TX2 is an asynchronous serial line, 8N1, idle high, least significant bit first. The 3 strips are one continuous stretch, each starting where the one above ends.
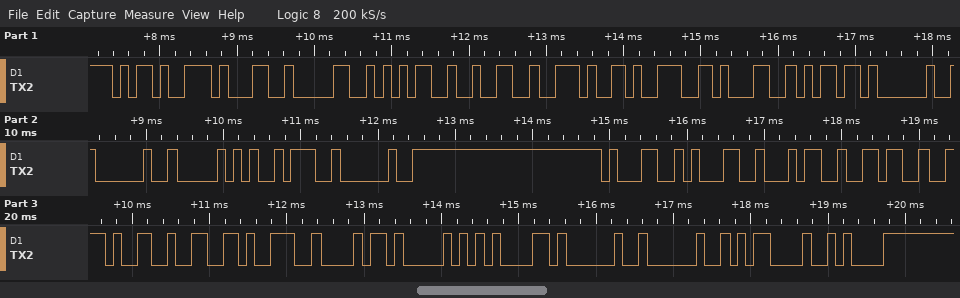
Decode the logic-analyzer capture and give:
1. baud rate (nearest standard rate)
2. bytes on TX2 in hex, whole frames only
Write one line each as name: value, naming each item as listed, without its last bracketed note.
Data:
baud rate: 9600 baud
bytes on TX2 in hex, whole frames only: 2D 31 30 35 32 2E 39 31 6D 20 20 50 3A 20 31 31 34 36 2E 32 39 68 50 61 20 20 0D 0A
